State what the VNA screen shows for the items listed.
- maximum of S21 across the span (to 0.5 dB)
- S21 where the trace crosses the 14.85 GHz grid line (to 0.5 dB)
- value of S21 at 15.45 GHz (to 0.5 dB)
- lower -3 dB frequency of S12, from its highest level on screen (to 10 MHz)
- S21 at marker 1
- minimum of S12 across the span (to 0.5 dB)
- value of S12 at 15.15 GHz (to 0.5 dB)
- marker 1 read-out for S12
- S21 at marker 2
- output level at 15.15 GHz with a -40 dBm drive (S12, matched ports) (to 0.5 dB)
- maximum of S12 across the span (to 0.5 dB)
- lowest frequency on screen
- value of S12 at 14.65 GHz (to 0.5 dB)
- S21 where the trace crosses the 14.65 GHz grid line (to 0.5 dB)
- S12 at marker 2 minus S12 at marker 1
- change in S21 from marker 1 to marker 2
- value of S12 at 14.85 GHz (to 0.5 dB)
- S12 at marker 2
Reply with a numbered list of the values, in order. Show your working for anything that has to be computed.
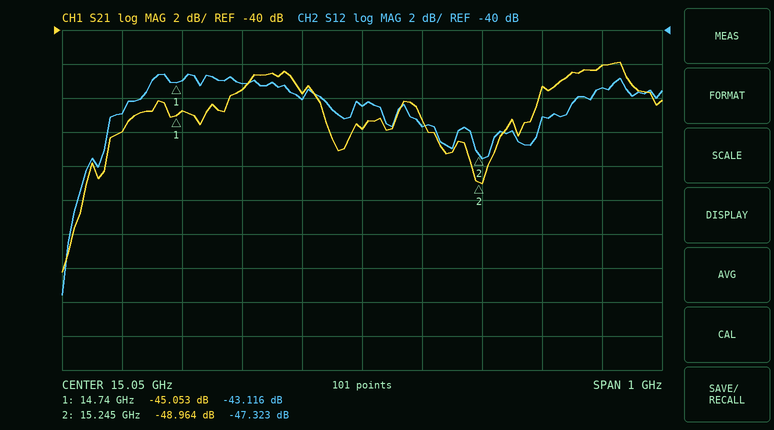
1. -42.0 dB
2. -43.5 dB
3. -42.0 dB
4. 14.63 GHz
5. -45.053 dB
6. -55.5 dB
7. -45.5 dB
8. -43.116 dB
9. -48.964 dB
10. -40 dBm + (-45.5 dB) = -85.5 dBm
11. -42.5 dB
12. 14.55 GHz
13. -45.0 dB
14. -46.0 dB
15. -47.323 − (-43.116) = -4.207 dB
16. -48.964 − (-45.053) = -3.911 dB
17. -43.0 dB
18. -47.323 dB
